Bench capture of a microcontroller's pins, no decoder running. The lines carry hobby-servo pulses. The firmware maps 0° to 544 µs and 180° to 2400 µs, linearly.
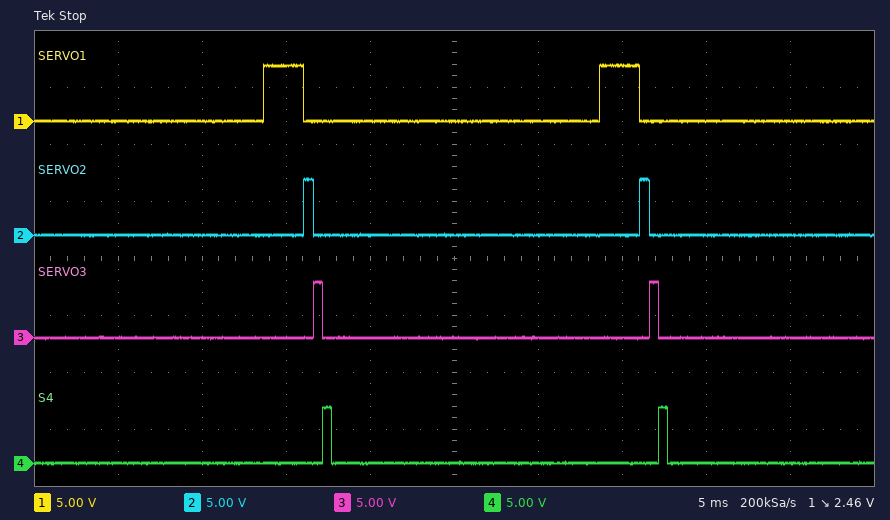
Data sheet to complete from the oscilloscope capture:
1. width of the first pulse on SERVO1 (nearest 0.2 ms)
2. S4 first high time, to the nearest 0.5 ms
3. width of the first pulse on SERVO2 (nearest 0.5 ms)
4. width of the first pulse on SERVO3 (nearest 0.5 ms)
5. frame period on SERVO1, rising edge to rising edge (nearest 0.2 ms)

2.4 ms
0.5 ms
0.5 ms
0.5 ms
20.0 ms
